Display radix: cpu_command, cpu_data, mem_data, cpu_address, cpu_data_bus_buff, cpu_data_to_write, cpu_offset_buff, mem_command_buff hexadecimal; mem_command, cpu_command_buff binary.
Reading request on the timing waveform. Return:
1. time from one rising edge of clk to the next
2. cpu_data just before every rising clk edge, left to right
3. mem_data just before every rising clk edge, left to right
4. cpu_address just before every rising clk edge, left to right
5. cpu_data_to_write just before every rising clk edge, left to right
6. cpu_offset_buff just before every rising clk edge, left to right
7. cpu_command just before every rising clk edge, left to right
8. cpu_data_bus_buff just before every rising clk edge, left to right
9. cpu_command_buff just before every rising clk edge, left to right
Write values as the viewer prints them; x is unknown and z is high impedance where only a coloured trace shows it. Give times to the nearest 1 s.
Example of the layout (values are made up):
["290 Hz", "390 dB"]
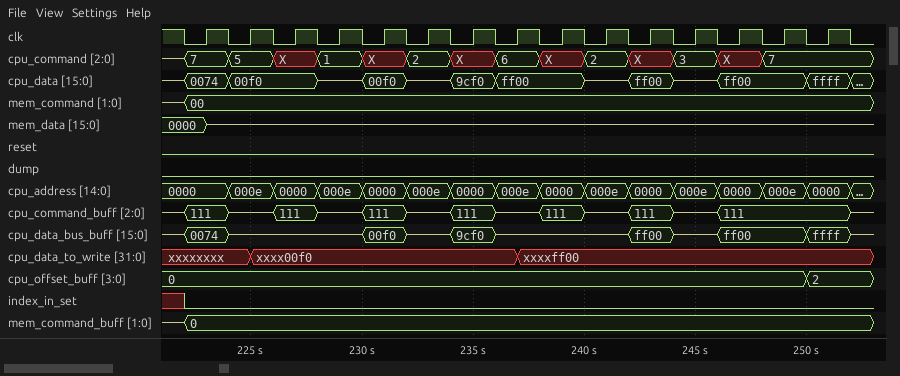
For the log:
["2 s", "0074, 00f0, 00f0, z, 00f0, z, 9cf0, ff00, ff00, z, ff00, z, ff00, ff00, ffff", "0000, z, z, z, z, z, z, z, z, z, z, z, z, z, z", "0000, 000e, 0000, 000e, 0000, 000e, 0000, 000e, 0000, 000e, 0000, 000e, 0000, 000e, 0000", "xxxxxxxx, xxxxxxxx, xxxx00f0, xxxx00f0, xxxx00f0, xxxx00f0, xxxx00f0, xxxx00f0, xxxxff00, xxxxff00, xxxxff00, xxxxff00, xxxxff00, xxxxff00, xxxxff00", "0, 0, 0, 0, 0, 0, 0, 0, 0, 0, 0, 0, 0, 0, 2", "7, 5, X, 1, X, 2, X, 6, X, 2, X, 3, X, 7, 7", "0074, z, z, z, 00f0, z, 9cf0, z, z, z, ff00, z, ff00, ff00, ffff", "111, z, 111, z, 111, z, 111, z, 111, z, 111, z, 111, 111, 111"]
